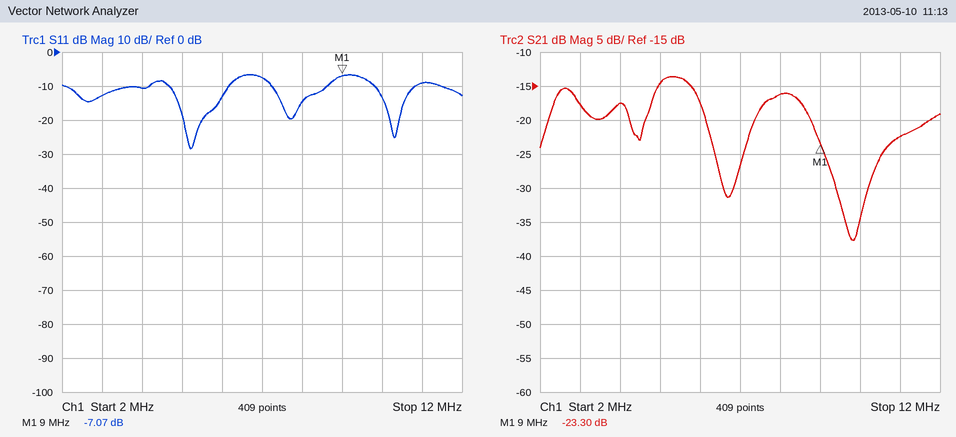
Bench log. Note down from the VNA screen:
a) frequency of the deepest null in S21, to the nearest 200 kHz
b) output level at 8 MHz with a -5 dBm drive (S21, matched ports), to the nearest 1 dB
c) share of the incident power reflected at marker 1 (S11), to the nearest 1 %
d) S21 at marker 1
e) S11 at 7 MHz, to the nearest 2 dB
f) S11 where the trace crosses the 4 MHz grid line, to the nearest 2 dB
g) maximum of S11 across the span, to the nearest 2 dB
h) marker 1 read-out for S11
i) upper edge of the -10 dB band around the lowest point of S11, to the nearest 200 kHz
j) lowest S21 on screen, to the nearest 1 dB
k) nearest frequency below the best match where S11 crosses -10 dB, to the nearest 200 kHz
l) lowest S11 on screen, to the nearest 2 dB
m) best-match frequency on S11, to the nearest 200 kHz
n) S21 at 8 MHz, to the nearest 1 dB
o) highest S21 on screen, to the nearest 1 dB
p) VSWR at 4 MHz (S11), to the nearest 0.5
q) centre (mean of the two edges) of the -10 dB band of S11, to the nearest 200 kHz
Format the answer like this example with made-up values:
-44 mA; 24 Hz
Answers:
9.8 MHz; -21 dBm; 20 %; -23.30 dB; -8 dB; -10 dB; -6 dB; -7.07 dB; 6.2 MHz; -38 dB; 4.6 MHz; -28 dB; 5.2 MHz; -16 dB; -14 dB; 2.0; 5.4 MHz
